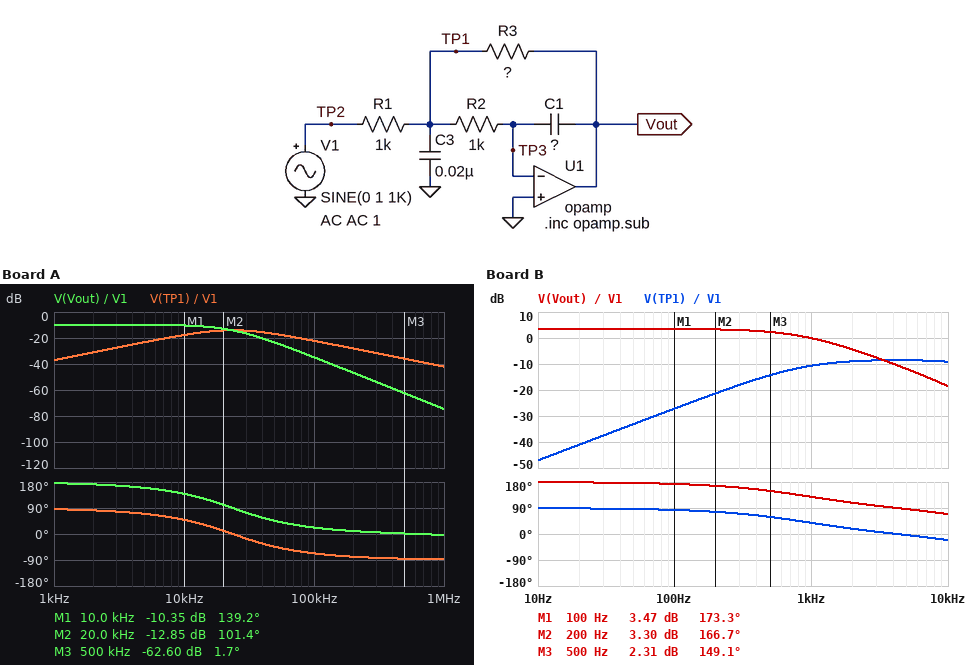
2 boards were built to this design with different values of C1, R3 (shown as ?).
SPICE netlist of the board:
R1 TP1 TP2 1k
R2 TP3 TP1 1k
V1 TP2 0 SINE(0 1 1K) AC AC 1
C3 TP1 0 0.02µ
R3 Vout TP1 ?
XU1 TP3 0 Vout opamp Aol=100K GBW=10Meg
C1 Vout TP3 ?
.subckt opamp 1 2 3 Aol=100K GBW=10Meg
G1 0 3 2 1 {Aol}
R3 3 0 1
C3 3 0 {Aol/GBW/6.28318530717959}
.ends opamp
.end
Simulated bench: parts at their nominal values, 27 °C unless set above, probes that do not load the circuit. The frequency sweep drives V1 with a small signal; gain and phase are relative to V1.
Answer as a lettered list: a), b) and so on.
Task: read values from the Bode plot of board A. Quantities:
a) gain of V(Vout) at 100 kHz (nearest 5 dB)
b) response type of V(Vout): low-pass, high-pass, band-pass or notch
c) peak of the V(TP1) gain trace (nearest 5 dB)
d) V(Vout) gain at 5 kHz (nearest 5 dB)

a) -35 dB
b) low-pass
c) -15 dB
d) -10 dB
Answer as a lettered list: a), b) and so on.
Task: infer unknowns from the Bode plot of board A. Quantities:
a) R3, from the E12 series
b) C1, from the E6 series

a) 330 Ω
b) 6.8 nF
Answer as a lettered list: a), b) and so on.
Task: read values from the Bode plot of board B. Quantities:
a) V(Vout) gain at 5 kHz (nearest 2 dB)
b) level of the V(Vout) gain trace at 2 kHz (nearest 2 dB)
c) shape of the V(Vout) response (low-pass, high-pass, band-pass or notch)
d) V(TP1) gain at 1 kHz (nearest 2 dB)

a) -12 dB
b) -4 dB
c) low-pass
d) -10 dB
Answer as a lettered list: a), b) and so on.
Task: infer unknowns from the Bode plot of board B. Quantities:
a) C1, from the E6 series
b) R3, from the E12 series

a) 47 nF
b) 1.5 kΩ
